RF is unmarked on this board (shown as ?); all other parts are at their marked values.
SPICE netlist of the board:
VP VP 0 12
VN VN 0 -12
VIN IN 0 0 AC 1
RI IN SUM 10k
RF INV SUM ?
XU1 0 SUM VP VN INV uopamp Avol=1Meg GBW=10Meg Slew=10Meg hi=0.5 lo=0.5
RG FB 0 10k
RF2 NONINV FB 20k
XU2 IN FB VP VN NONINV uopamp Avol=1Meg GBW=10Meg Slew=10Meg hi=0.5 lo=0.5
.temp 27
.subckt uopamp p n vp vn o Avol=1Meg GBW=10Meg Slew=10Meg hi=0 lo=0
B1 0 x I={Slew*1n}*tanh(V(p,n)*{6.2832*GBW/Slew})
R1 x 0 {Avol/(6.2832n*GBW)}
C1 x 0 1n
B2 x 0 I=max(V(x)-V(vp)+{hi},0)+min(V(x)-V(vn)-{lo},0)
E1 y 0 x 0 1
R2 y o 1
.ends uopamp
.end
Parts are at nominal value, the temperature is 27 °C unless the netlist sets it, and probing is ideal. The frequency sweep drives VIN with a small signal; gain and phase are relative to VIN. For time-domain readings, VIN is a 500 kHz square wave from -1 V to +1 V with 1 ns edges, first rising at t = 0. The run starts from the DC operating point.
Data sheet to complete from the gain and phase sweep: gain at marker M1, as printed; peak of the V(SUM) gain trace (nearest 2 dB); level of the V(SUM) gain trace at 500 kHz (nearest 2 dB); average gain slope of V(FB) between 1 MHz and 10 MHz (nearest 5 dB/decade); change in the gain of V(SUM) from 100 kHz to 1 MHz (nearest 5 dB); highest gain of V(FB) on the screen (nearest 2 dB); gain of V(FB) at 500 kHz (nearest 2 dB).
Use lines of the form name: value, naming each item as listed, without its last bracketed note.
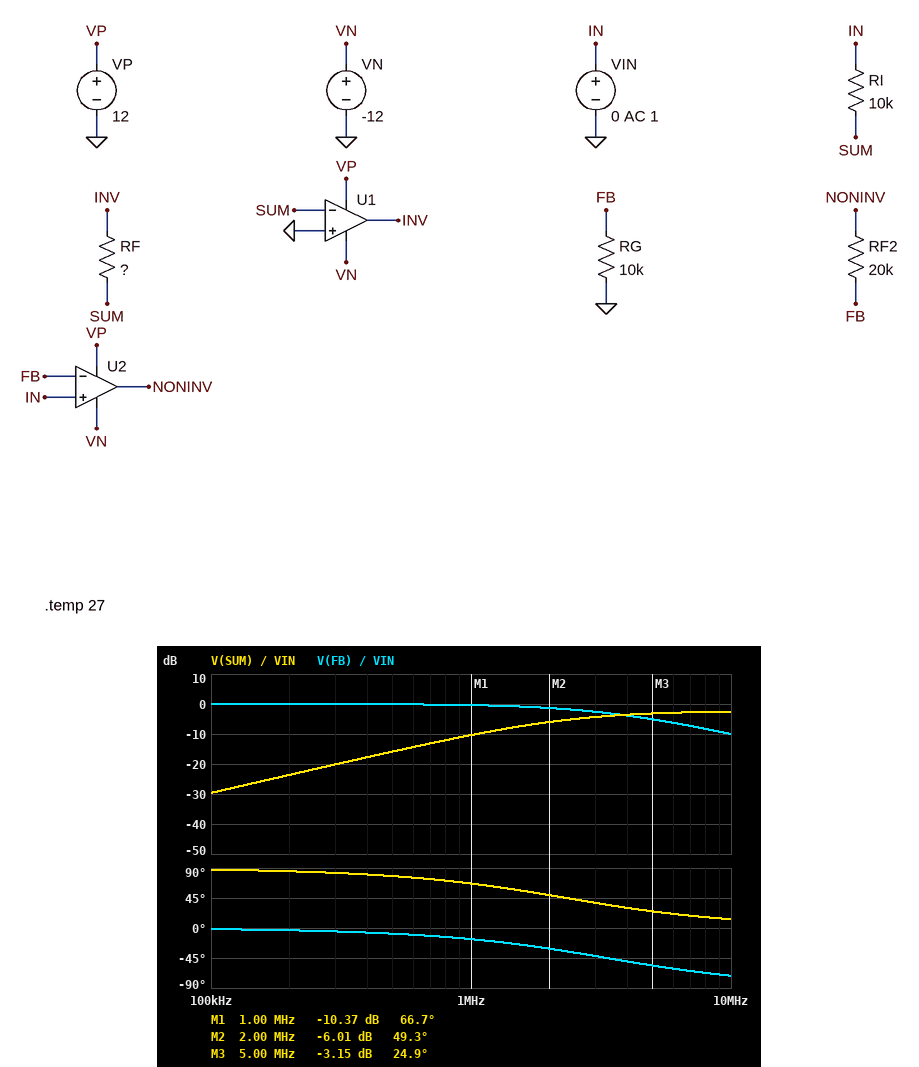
gain at marker M1, as printed: -10.37 dB
peak of the V(SUM) gain trace: -2 dB
level of the V(SUM) gain trace at 500 kHz: -16 dB
average gain slope of V(FB) between 1 MHz and 10 MHz: -10 dB/decade
change in the gain of V(SUM) from 100 kHz to 1 MHz: 20 dB
highest gain of V(FB) on the screen: 0 dB
gain of V(FB) at 500 kHz: 0 dB
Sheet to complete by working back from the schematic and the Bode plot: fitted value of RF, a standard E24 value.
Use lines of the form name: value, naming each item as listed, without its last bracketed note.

fitted value of RF, a standard E24 value: 33 kΩ
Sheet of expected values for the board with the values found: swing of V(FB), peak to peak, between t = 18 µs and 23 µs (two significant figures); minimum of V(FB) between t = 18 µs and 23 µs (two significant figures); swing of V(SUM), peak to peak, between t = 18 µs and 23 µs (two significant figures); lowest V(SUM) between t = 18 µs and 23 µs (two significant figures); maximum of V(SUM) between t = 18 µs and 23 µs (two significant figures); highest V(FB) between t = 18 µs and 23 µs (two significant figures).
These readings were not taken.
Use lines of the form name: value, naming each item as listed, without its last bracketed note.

swing of V(FB), peak to peak, between t = 18 µs and 23 µs: 2.0 V
minimum of V(FB) between t = 18 µs and 23 µs: -1.0 V
swing of V(SUM), peak to peak, between t = 18 µs and 23 µs: 3.1 V
lowest V(SUM) between t = 18 µs and 23 µs: -1.5 V
maximum of V(SUM) between t = 18 µs and 23 µs: 1.5 V
highest V(FB) between t = 18 µs and 23 µs: 1.0 V
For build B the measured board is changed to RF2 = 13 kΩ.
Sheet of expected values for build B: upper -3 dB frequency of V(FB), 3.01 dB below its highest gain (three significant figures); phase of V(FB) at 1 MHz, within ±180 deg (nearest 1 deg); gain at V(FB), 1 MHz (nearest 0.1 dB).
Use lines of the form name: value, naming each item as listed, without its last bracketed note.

upper -3 dB frequency of V(FB), 3.01 dB below its highest gain: 4.35 MHz
phase of V(FB) at 1 MHz, within ±180 deg: -13 deg
gain at V(FB), 1 MHz: -0.2 dB
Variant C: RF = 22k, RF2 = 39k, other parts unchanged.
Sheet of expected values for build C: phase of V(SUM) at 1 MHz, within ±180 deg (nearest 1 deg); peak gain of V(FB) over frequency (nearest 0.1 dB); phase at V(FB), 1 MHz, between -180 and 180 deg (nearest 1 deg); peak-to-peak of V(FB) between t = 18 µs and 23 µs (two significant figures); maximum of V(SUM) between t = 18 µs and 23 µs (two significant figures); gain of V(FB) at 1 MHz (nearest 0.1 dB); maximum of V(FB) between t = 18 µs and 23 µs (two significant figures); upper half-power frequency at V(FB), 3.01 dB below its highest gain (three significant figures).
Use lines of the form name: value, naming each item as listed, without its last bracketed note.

phase of V(SUM) at 1 MHz, within ±180 deg: 72 deg
peak gain of V(FB) over frequency: 0 dB
phase at V(FB), 1 MHz, between -180 and 180 deg: -26 deg
peak-to-peak of V(FB) between t = 18 µs and 23 µs: 1.9 V
maximum of V(SUM) between t = 18 µs and 23 µs: 1.4 V
gain of V(FB) at 1 MHz: -0.9 dB
maximum of V(FB) between t = 18 µs and 23 µs: 950 mV
upper half-power frequency at V(FB), 3.01 dB below its highest gain: 2.04 MHz
